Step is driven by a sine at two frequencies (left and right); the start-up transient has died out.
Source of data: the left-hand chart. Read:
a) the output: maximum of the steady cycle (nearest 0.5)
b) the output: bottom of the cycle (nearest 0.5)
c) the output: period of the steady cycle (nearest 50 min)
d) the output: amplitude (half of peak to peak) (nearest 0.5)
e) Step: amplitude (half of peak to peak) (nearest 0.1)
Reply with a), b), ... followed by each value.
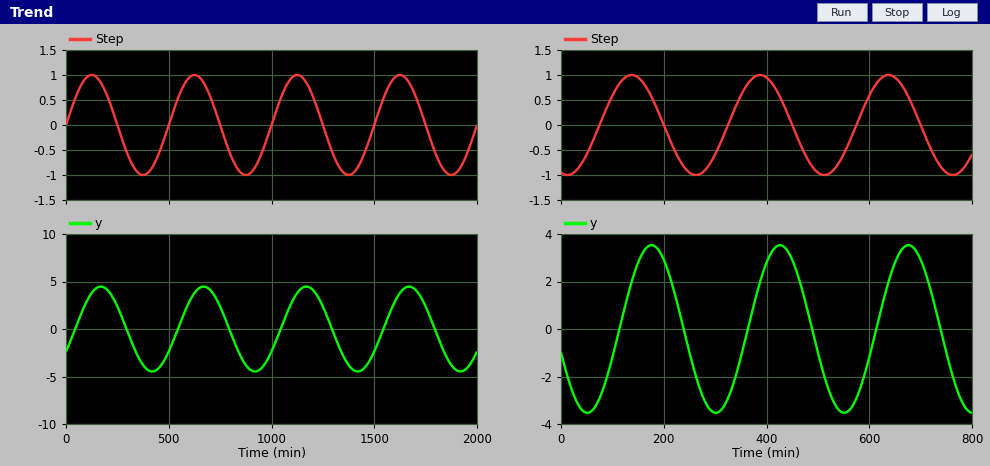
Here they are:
a) 4.5
b) -4.5
c) 500 min
d) 4.5
e) 1.0
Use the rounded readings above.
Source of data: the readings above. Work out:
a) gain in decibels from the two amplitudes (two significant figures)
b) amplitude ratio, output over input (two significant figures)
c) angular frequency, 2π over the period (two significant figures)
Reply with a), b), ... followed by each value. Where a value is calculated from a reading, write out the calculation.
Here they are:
a) 20 log10(4.5 / 1) = 13 dB
b) 4.5 / 1 = 4.5
c) 2π / 500 = 0.013 rad/min
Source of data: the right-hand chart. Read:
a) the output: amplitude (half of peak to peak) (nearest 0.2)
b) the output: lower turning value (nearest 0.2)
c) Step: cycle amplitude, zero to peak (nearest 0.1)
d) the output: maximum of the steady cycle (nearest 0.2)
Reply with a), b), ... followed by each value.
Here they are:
a) 3.6
b) -3.6
c) 1.0
d) 3.6
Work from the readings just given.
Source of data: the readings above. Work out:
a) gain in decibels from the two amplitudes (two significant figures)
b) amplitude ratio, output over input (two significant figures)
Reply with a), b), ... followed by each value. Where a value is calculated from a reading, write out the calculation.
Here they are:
a) 20 log10(3.6 / 1) = 11 dB
b) 3.6 / 1 = 3.6
